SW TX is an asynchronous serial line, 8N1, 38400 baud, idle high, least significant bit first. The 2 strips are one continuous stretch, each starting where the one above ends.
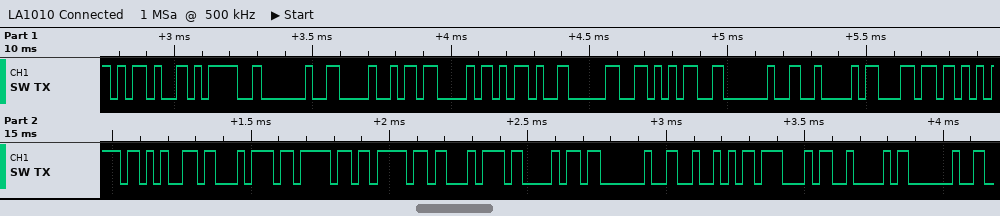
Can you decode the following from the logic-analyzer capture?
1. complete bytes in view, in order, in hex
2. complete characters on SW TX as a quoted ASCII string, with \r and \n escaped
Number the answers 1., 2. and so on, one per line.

1. 2D 3D 20 48 43 2D 30 35 20 42 6C 75 65 74 6F 6F 74 68 20 52 47 42 20
2. "-= HC-05 Bluetooth RGB "
